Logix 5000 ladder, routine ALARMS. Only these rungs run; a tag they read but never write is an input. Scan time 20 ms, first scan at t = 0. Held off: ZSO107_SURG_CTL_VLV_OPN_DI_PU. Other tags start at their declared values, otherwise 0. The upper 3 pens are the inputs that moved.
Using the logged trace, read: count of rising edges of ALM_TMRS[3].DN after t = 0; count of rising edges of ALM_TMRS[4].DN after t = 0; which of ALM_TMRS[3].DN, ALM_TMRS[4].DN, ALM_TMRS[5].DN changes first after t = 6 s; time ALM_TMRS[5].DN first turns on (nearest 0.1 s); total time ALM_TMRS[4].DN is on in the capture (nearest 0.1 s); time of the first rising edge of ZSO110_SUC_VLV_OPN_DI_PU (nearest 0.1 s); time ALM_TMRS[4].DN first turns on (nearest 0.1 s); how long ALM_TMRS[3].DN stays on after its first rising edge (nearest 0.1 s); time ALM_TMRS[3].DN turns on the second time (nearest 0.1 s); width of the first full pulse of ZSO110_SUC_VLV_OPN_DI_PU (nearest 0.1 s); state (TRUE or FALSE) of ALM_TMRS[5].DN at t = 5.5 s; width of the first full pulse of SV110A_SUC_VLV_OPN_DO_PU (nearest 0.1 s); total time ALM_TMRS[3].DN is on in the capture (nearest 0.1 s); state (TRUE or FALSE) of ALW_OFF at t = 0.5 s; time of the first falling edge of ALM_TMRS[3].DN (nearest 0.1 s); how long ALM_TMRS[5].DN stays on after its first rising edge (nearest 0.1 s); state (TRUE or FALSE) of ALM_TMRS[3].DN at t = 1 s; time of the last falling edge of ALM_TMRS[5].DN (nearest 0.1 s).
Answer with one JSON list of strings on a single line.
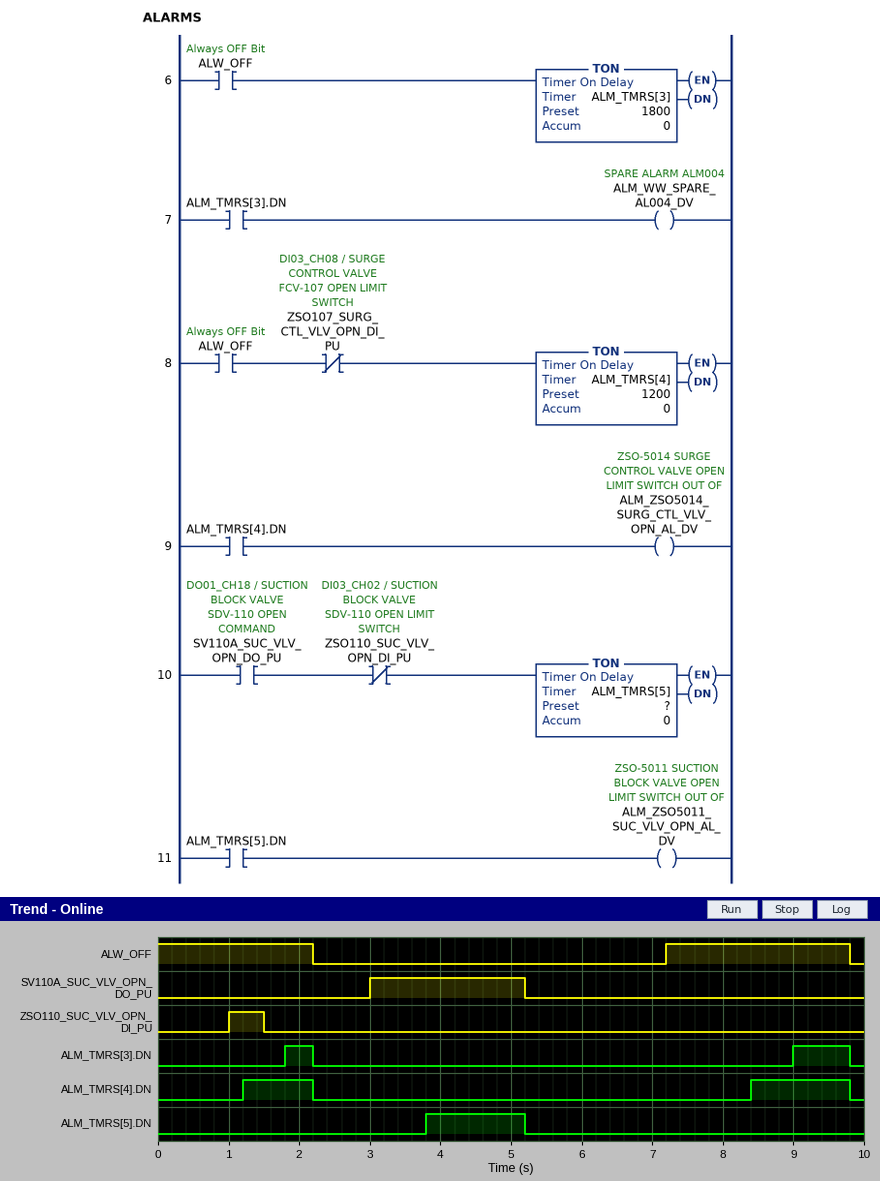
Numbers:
["2", "2", "ALM_TMRS[4].DN", "3.8 s", "2.4 s", "1.0 s", "1.2 s", "0.4 s", "9.0 s", "0.5 s", "FALSE", "2.2 s", "1.2 s", "TRUE", "2.2 s", "1.4 s", "FALSE", "5.2 s"]
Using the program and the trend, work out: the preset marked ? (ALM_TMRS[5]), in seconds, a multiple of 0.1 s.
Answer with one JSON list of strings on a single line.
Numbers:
["0.8 s"]
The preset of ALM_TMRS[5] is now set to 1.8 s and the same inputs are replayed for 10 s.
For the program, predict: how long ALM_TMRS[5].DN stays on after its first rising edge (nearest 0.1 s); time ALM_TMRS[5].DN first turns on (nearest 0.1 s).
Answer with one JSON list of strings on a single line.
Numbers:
["0.4 s", "4.8 s"]
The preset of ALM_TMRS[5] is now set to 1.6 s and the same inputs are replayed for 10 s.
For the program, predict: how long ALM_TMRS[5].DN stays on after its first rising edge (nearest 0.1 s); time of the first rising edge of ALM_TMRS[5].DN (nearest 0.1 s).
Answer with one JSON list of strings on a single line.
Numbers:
["0.6 s", "4.6 s"]
